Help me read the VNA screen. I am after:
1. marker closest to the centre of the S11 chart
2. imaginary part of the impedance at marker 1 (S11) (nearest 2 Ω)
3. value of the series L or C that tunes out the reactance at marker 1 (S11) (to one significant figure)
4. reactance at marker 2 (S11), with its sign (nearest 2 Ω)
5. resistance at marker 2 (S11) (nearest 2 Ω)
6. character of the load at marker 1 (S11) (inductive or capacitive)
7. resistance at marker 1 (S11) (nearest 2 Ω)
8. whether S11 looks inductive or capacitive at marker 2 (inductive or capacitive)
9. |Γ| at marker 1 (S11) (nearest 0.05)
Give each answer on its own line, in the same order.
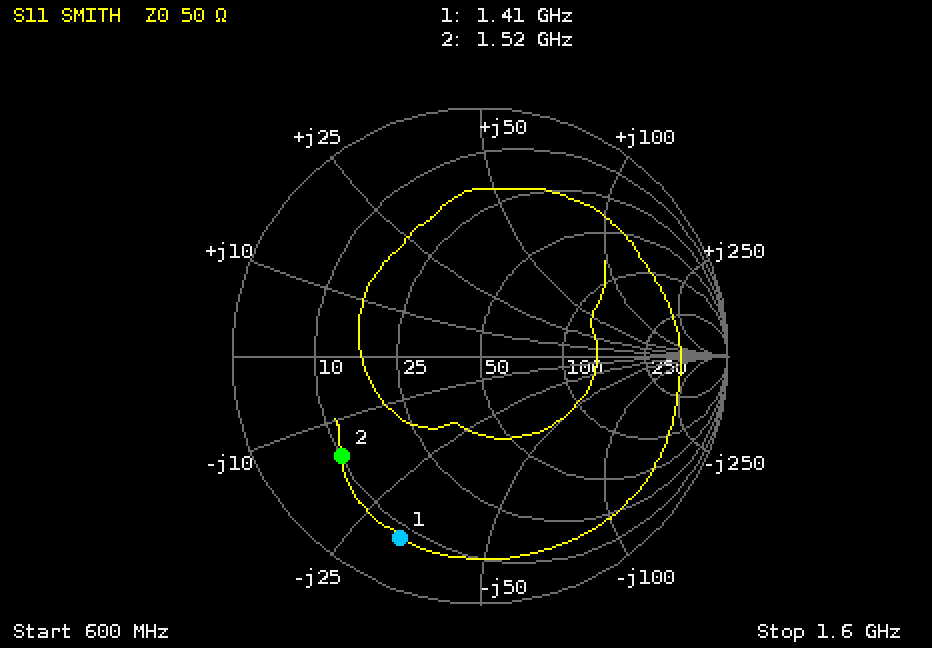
marker 2
-32 Ω
4 nH
-16 Ω
10 Ω
capacitive
8 Ω
capacitive
0.80
